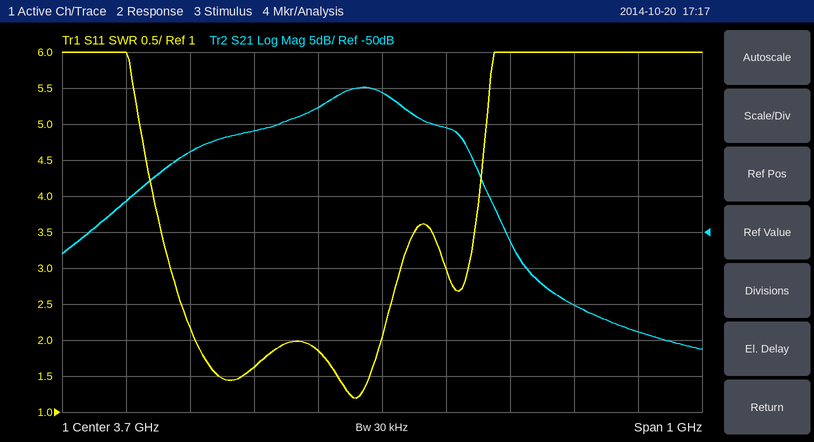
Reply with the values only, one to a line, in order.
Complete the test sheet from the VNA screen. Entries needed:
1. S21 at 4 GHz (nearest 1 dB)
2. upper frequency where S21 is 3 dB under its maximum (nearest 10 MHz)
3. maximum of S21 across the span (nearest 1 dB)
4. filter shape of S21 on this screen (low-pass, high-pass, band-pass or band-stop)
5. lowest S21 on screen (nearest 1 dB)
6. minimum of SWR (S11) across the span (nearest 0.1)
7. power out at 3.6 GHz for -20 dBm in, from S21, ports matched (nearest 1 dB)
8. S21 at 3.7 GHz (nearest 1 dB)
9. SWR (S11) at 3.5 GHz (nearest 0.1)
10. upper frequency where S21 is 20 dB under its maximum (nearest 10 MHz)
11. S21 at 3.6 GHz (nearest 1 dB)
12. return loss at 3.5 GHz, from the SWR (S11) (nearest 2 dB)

-60 dB
3.74 GHz
-30 dB
band-pass
-66 dB
1.2
-53 dBm
-31 dB
1.6
3.89 GHz
-33 dB
12 dB
